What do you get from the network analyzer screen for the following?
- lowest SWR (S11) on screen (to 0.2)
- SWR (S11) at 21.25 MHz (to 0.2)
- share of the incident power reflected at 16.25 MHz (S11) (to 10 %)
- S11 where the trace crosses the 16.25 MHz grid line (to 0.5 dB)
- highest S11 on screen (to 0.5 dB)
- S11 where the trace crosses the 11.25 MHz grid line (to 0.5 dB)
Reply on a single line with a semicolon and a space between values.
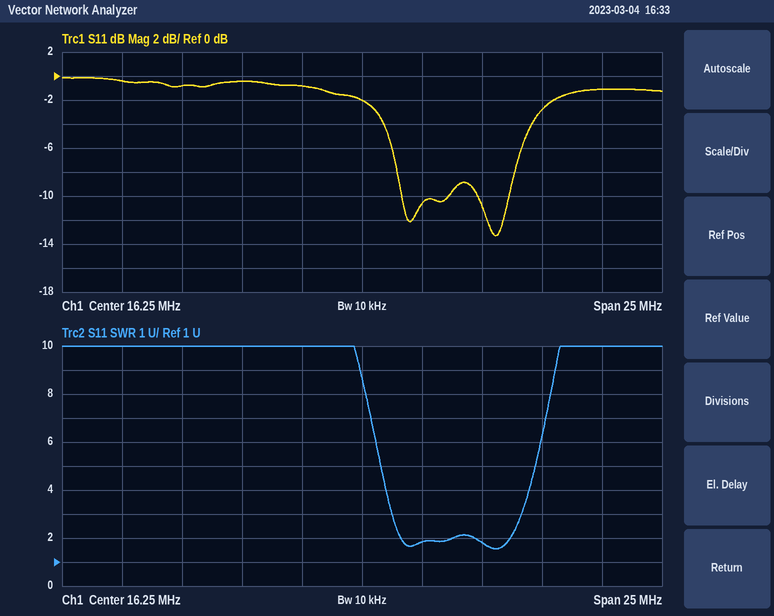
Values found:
1.6; 1.8; 60 %; -2.0 dB; 0.0 dB; -0.5 dB
